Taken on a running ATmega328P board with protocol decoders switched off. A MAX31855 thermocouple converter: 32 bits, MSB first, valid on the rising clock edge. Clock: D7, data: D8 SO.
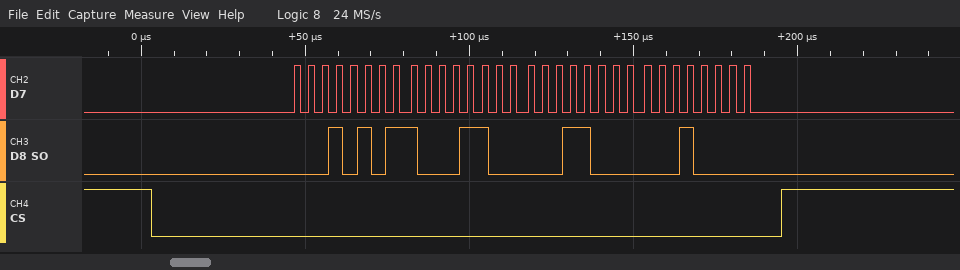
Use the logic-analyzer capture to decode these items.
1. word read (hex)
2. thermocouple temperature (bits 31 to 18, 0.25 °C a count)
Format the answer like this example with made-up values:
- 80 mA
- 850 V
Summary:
- 0x158C1810
- 344.75 °C
